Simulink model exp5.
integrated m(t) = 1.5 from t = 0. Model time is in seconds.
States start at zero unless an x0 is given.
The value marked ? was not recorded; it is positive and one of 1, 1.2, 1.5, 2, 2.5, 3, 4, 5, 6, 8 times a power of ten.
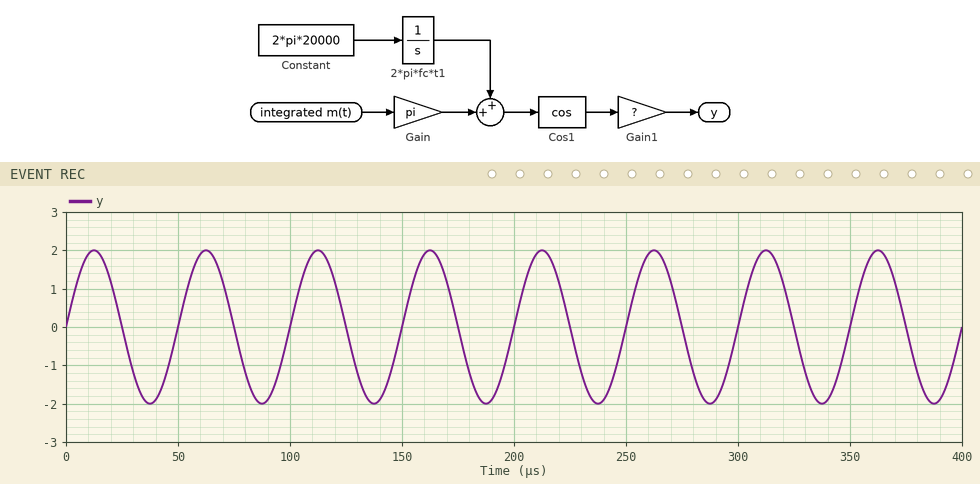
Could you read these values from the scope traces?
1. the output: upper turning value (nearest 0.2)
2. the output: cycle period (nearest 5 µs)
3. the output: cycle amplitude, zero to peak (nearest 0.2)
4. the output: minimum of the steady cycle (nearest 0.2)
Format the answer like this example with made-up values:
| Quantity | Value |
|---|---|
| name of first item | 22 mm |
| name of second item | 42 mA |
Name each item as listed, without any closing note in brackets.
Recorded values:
| Quantity | Value |
|---|---|
| the output: upper turning value | 2.0 |
| the output: cycle period | 50 µs |
| the output: cycle amplitude, zero to peak | 2.0 |
| the output: minimum of the steady cycle | -2.0 |
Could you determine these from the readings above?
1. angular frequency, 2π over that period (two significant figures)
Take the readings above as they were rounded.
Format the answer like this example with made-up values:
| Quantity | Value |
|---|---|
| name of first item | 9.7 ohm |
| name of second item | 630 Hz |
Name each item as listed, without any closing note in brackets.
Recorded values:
| Quantity | Value |
|---|---|
| angular frequency, 2π over that period | 0.13 rad/µs |
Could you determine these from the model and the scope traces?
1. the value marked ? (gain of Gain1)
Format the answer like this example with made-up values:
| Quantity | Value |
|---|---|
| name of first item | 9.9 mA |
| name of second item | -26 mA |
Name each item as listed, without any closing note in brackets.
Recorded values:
| Quantity | Value |
|---|---|
| the value marked ? | 2 |
